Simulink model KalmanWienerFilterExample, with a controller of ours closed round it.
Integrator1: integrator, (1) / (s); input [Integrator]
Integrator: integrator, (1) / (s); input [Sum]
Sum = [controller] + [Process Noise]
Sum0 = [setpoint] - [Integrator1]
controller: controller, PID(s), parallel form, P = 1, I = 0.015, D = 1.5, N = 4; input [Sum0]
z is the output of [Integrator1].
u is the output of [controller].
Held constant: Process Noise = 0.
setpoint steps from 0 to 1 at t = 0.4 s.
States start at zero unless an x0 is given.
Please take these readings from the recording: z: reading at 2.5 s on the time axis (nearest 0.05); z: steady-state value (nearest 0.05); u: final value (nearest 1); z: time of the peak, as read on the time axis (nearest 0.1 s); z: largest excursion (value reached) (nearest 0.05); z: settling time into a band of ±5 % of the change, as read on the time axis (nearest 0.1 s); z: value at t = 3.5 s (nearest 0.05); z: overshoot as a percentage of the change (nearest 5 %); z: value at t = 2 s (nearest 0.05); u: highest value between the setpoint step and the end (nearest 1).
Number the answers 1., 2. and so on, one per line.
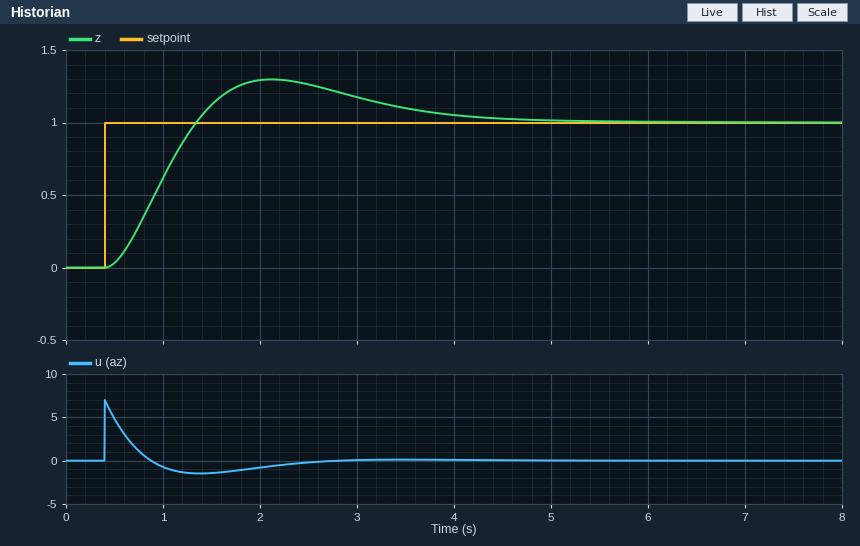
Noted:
1. 1.25
2. 1.00
3. 0
4. 2.1 s
5. 1.30
6. 4.0 s
7. 1.10
8. 30 %
9. 1.30
10. 7
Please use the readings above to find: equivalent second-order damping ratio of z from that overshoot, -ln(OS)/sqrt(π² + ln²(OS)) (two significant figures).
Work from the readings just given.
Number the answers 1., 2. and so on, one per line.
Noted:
1. 0.36
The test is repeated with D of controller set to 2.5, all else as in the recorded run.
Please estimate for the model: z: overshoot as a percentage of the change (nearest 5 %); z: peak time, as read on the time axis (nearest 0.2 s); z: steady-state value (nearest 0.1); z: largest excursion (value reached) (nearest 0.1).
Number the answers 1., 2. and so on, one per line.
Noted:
1. 25 %
2. 1.6 s
3. 1.0
4. 1.2
